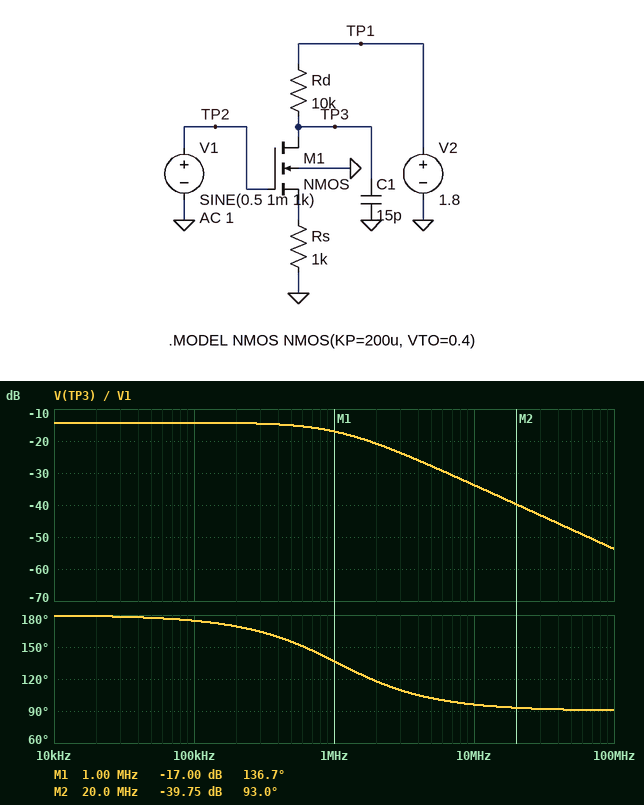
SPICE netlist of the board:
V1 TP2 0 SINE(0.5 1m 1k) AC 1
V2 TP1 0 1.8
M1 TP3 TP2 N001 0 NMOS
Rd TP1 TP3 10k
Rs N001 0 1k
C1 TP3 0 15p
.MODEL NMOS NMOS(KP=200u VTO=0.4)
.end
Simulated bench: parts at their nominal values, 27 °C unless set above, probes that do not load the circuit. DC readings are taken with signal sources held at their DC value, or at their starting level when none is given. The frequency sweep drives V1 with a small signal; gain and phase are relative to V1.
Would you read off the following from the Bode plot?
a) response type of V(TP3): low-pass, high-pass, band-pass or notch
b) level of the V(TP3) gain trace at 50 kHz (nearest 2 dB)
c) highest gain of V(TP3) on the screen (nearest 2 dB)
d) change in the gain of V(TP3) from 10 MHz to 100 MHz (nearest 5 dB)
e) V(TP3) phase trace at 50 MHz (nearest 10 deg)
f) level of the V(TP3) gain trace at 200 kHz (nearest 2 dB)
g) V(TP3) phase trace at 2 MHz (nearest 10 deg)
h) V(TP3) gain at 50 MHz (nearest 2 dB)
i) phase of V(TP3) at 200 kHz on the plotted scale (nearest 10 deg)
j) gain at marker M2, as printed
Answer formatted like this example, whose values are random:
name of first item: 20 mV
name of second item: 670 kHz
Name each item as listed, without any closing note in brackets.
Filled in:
response type of V(TP3): low-pass, high-pass, band-pass or notch: low-pass
level of the V(TP3) gain trace at 50 kHz: -14 dB
highest gain of V(TP3) on the screen: -14 dB
change in the gain of V(TP3) from 10 MHz to 100 MHz: -20 dB
V(TP3) phase trace at 50 MHz: 90 deg
level of the V(TP3) gain trace at 200 kHz: -14 dB
V(TP3) phase trace at 2 MHz: 120 deg
V(TP3) gain at 50 MHz: -48 dB
phase of V(TP3) at 200 kHz on the plotted scale: 170 deg
gain at marker M2, as printed: -39.75 dB
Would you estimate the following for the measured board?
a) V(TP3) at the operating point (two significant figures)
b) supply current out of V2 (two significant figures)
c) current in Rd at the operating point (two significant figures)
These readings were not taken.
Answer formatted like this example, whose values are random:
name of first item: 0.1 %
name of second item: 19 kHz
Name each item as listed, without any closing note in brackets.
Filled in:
V(TP3) at the operating point: 1.8 V
supply current out of V2: 980 nA
current in Rd at the operating point: 980 nA
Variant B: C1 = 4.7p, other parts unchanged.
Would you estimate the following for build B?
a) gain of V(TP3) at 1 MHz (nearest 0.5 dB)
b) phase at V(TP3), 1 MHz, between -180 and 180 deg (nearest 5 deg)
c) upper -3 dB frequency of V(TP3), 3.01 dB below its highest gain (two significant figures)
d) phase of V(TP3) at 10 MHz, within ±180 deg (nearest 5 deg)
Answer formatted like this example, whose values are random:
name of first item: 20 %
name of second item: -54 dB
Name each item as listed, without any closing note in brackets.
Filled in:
gain of V(TP3) at 1 MHz: -14.5 dB
phase at V(TP3), 1 MHz, between -180 and 180 deg: 165 deg
upper -3 dB frequency of V(TP3), 3.01 dB below its highest gain: 3.4 MHz
phase of V(TP3) at 10 MHz, within ±180 deg: 110 deg
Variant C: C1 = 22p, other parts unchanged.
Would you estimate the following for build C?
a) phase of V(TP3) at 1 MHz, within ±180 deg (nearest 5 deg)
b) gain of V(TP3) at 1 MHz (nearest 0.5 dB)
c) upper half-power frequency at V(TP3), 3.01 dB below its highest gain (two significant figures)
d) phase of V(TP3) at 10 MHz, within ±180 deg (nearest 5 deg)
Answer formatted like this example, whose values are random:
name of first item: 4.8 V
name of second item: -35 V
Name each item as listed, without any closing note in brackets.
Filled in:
phase of V(TP3) at 1 MHz, within ±180 deg: 125 deg
gain of V(TP3) at 1 MHz: -19.0 dB
upper half-power frequency at V(TP3), 3.01 dB below its highest gain: 720 kHz
phase of V(TP3) at 10 MHz, within ±180 deg: 95 deg
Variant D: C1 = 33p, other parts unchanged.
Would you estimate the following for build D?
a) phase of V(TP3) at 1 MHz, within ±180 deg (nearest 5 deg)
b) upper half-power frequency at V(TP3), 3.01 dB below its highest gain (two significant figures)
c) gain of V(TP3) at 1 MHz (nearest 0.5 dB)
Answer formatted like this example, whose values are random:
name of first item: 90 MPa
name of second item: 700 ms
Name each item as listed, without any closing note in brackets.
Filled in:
phase of V(TP3) at 1 MHz, within ±180 deg: 115 deg
upper half-power frequency at V(TP3), 3.01 dB below its highest gain: 480 kHz
gain of V(TP3) at 1 MHz: -21.5 dB
